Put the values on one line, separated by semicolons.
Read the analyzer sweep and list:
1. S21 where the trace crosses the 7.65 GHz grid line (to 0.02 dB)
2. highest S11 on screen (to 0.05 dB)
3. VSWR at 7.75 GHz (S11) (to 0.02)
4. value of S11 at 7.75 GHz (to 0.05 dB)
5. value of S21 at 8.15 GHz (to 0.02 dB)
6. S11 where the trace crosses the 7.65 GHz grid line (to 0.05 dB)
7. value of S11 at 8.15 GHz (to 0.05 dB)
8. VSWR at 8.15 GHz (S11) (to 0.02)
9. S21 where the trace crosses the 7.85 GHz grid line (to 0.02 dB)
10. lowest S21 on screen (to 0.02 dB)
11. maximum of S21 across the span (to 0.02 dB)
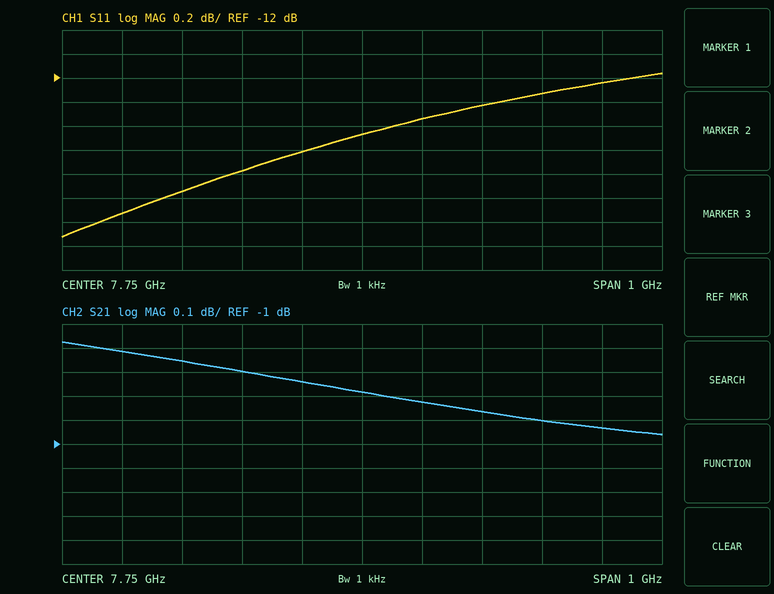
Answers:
-0.74 dB; -11.95 dB; 1.62; -12.45 dB; -0.94 dB; -12.60 dB; -12.05 dB; 1.66; -0.82 dB; -0.96 dB; -0.58 dB
